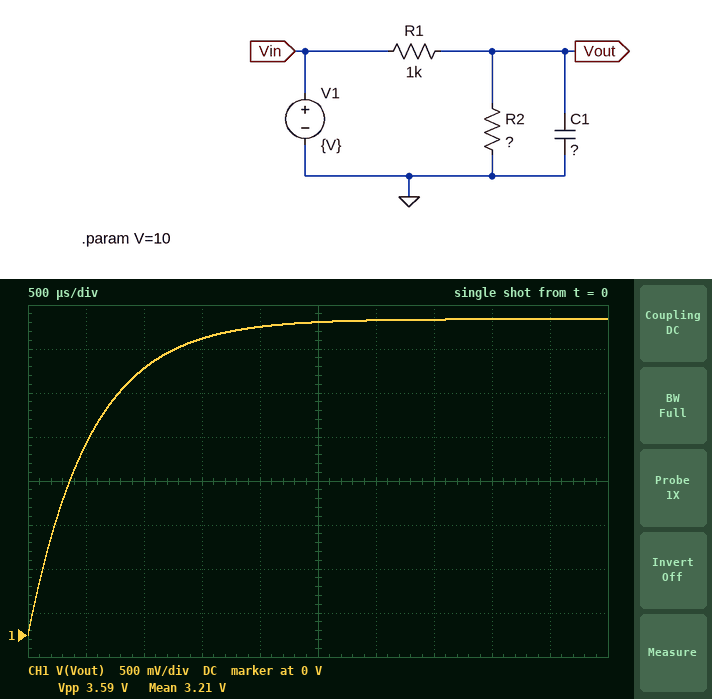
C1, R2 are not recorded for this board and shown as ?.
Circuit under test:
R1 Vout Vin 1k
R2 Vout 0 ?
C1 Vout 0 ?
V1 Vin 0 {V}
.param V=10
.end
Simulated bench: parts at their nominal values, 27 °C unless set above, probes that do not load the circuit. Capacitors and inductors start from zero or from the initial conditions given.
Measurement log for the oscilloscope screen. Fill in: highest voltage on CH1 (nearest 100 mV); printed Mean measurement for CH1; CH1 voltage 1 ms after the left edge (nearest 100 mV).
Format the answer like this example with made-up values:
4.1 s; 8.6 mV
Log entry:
3.6 V; 3.21 V; 3.0 V
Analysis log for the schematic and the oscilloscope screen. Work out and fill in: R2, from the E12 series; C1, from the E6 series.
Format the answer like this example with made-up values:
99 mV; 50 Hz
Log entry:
560 Ω; 1.5 µF
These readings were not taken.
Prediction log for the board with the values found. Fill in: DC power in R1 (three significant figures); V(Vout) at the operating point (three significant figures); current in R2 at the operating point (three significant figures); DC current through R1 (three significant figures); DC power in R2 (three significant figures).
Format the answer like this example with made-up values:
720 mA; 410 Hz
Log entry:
41.1 mW; 3.59 V; 6.41 mA; 6.41 mA; 23.0 mW
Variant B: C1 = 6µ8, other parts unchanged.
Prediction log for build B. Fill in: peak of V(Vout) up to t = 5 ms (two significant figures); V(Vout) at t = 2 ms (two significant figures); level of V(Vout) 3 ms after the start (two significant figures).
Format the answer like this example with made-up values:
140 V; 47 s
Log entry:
3.1 V; 2.0 V; 2.5 V
